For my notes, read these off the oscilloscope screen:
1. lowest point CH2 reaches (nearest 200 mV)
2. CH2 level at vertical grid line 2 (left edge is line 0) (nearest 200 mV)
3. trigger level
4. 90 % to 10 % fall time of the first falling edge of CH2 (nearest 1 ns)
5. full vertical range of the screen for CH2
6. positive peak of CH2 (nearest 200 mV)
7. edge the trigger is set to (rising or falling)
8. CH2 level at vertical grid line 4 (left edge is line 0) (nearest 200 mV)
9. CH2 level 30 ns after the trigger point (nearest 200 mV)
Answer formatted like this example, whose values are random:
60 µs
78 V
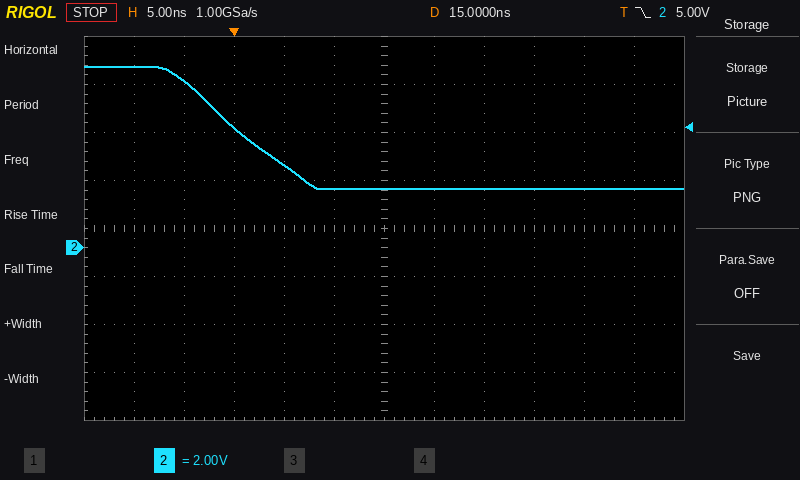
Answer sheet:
2.4 V
7.0 V
5.00 V
12 ns
16 V
7.6 V
falling
3.4 V
2.4 V
